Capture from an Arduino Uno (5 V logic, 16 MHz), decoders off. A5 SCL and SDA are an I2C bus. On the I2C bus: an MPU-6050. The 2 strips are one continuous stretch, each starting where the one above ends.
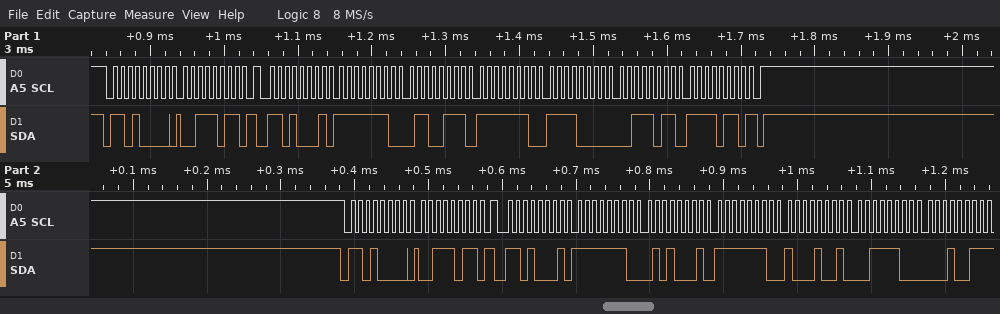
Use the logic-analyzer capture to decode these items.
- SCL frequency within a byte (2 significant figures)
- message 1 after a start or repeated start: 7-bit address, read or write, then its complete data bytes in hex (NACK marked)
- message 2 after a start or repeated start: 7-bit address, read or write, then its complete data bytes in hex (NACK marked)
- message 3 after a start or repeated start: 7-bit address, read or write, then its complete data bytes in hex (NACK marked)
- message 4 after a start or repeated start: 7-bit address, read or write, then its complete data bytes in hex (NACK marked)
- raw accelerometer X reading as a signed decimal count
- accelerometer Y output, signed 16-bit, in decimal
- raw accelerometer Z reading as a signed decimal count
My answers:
100 kHz
0x68 write: 3B
0x68 read: FE 67 FE F0 3B F6 NACK
0x68 write: 3B
0x68 read: FE 51 FE 89 3C 13 NACK
-409
-272
15350
